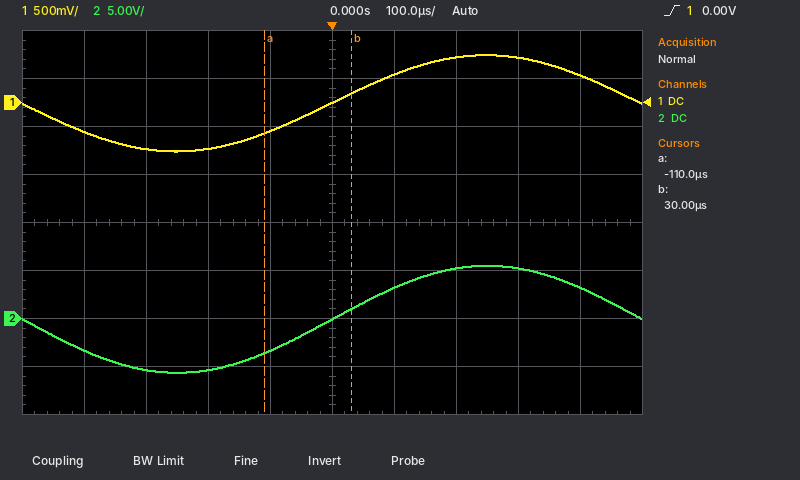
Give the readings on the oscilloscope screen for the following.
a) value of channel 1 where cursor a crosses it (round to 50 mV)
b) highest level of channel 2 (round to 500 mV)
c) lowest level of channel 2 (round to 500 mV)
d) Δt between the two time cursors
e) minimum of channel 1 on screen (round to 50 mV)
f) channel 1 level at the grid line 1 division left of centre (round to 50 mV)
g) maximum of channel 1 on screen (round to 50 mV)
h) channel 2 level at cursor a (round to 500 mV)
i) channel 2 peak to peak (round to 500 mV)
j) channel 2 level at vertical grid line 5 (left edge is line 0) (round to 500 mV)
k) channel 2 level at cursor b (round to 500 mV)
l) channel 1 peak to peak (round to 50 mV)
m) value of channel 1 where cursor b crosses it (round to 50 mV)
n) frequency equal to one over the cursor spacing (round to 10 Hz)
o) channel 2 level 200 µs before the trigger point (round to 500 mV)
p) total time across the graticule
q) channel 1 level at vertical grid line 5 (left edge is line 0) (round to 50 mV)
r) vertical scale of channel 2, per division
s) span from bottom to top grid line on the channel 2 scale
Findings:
-300 mV
5.5 V
-5.5 V
140 µs
-500 mV
-300 mV
500 mV
-3.5 V
11.0 V
0.0 V
1.0 V
1.00 V
100 mV
7.14 kHz
-5.5 V
1 ms
0 mV
5 V
40 V
